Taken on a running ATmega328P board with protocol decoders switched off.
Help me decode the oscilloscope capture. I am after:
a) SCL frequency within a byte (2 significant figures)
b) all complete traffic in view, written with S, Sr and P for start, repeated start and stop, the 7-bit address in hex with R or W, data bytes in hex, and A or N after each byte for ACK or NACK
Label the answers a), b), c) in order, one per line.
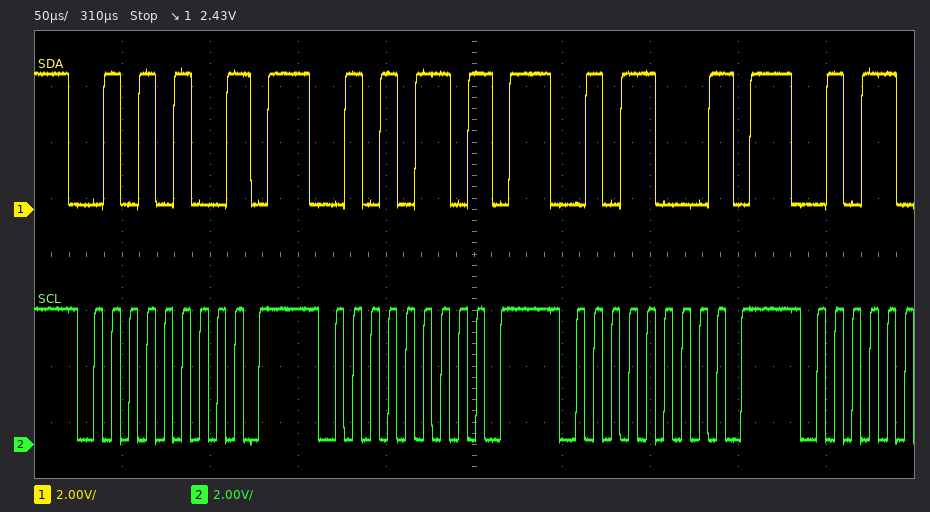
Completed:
a) 100 kHz
b) S 2AW N P S 2BW N P S 2CW N P
